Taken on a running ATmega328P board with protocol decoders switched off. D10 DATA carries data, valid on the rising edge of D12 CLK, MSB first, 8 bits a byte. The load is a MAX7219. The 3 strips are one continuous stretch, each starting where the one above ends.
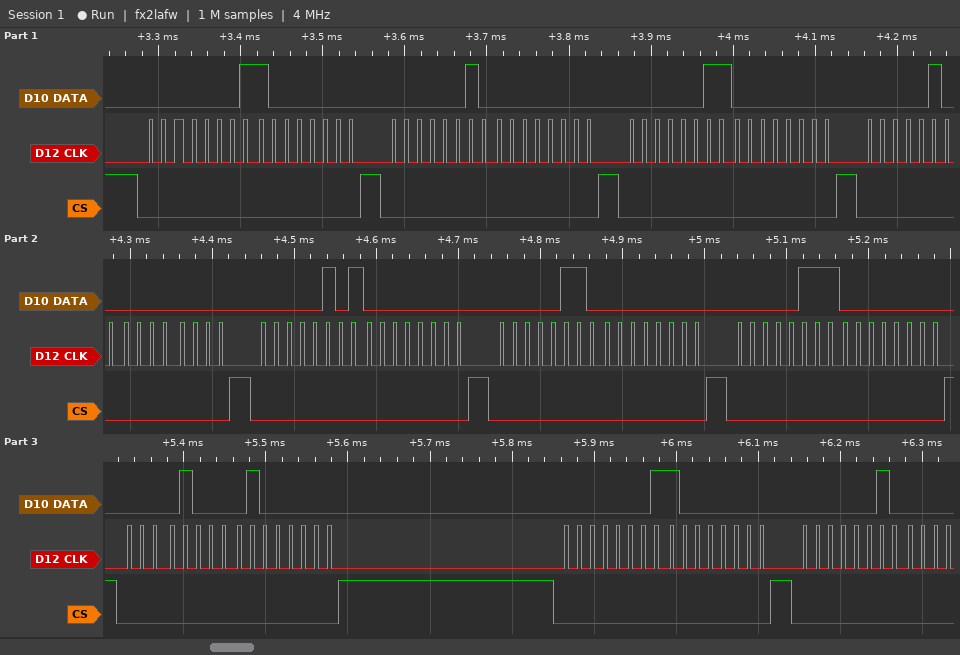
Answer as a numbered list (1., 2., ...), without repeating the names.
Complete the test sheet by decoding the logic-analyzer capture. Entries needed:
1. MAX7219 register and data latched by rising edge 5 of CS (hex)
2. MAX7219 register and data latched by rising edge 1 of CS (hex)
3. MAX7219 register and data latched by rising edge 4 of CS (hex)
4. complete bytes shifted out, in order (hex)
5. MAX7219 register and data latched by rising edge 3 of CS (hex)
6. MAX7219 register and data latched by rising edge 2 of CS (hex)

1. register 0x5, data 0x00
2. register 0x1, data 0x80
3. register 0x4, data 0x00
4. 01 80 02 00 03 00 04 00 05 00 06 00 07 00 08 40 01 80 02
5. register 0x3, data 0x00
6. register 0x2, data 0x00
